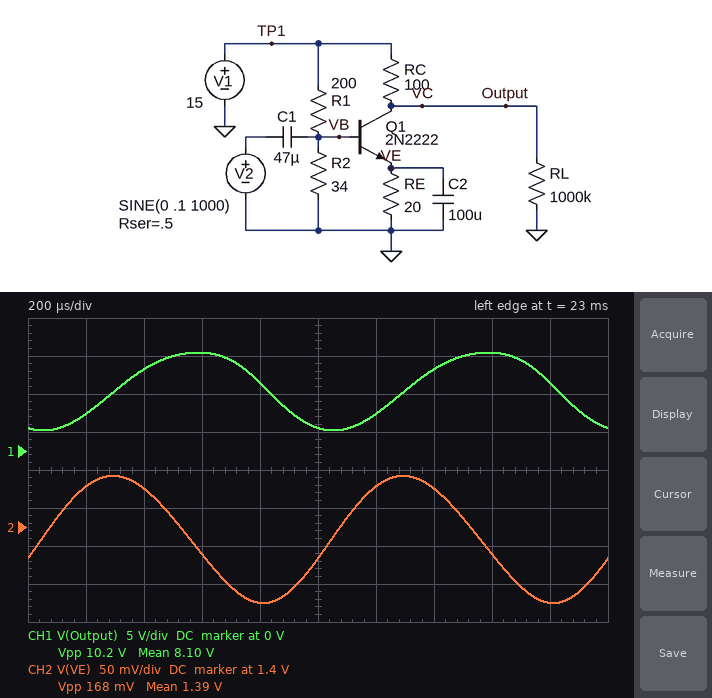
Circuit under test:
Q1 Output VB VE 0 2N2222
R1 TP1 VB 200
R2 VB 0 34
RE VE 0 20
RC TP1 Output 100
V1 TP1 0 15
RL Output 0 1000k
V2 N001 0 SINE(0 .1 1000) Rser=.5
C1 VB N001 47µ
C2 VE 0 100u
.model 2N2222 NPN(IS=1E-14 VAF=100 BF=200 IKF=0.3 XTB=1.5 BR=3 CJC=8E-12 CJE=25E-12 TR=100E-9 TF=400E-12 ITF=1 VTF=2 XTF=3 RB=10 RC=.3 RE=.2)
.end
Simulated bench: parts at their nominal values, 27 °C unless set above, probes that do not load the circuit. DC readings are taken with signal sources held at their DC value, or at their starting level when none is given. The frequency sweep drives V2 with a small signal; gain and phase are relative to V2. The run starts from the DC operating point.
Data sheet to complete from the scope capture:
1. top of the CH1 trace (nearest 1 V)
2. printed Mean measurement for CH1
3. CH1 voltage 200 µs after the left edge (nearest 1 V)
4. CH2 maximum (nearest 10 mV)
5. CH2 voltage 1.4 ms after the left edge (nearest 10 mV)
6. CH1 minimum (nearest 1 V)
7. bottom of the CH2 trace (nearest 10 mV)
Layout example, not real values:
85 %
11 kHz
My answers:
13 V
8.10 V
5 V
1.47 V
1.45 V
3 V
1.30 V
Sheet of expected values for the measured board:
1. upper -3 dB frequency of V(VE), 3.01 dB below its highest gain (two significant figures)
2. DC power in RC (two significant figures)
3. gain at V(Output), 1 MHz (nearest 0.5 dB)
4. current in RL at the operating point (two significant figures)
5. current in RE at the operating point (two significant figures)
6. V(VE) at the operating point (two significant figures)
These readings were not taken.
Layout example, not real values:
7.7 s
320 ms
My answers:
2.5 kHz
470 mW
42.5 dB
8.1 µA
69 mA
1.4 V
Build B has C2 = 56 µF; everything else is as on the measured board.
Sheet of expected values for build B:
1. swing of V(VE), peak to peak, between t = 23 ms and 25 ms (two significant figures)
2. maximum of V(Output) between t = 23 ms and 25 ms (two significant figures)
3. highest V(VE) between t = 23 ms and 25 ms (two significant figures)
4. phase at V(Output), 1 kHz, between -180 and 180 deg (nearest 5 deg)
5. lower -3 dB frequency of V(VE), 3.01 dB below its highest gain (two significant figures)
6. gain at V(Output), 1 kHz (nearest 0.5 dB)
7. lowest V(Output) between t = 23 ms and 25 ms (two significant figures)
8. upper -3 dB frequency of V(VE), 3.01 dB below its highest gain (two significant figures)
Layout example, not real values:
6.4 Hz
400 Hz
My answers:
180 mV
11 V
1.5 V
-105 deg
110 Hz
30.0 dB
4.9 V
4.2 kHz
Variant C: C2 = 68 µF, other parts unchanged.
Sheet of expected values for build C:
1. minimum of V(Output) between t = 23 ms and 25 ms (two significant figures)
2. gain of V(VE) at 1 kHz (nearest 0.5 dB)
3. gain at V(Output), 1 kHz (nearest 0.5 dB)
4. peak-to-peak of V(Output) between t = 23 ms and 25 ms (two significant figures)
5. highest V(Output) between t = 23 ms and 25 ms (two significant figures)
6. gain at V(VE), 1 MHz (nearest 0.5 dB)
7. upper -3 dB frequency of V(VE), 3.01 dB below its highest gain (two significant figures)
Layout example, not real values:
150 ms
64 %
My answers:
4.3 V
-1.0 dB
31.5 dB
7.5 V
12 V
-50.0 dB
3.5 kHz
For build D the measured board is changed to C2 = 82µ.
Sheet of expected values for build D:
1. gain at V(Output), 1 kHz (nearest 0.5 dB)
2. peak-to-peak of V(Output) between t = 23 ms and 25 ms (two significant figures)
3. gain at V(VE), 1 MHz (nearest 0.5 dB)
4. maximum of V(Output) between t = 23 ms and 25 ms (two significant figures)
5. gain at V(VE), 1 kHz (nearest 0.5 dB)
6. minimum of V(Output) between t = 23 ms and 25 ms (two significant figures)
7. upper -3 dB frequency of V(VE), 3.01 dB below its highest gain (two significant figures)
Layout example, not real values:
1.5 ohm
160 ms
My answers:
33.0 dB
8.8 V
-52.0 dB
12 V
-1.0 dB
3.6 V
3.0 kHz
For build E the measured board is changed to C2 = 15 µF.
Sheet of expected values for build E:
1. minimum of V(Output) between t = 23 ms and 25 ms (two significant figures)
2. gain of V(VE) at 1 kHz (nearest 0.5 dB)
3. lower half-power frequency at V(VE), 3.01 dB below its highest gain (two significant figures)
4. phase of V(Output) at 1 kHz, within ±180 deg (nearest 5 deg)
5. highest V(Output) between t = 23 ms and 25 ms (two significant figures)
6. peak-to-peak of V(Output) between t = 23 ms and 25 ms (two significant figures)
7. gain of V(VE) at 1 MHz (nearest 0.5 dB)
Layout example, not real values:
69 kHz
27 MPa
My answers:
7.1 V
-0.5 dB
110 Hz
-115 deg
9.1 V
2.0 V
-37.0 dB
